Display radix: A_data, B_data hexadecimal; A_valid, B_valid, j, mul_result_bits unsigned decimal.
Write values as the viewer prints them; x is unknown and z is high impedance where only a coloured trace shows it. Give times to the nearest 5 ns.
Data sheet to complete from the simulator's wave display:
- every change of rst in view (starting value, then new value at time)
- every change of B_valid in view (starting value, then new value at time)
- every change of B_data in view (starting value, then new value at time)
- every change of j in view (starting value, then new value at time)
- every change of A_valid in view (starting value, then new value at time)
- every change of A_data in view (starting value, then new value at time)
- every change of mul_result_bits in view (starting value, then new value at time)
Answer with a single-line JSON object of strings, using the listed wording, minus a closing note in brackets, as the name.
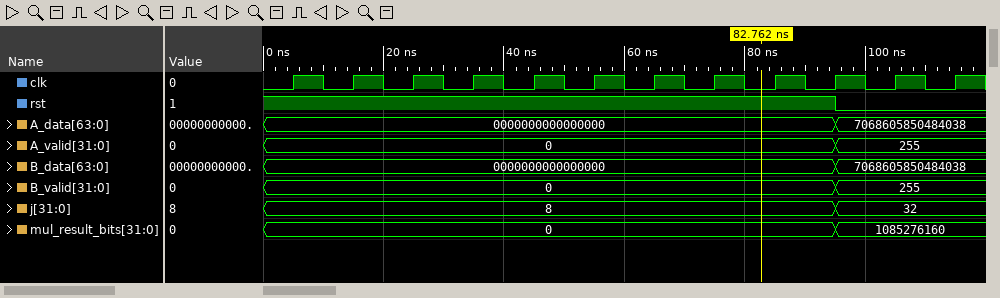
{"every change of rst in view": "1, 0 at 95 ns", "every change of B_valid in view": "0, 255 at 95 ns", "every change of B_data in view": "0000000000000000, 7068605850484038 at 95 ns", "every change of j in view": "8, 32 at 95 ns", "every change of A_valid in view": "0, 255 at 95 ns", "every change of A_data in view": "0000000000000000, 7068605850484038 at 95 ns", "every change of mul_result_bits in view": "0, 1085276160 at 95 ns"}
